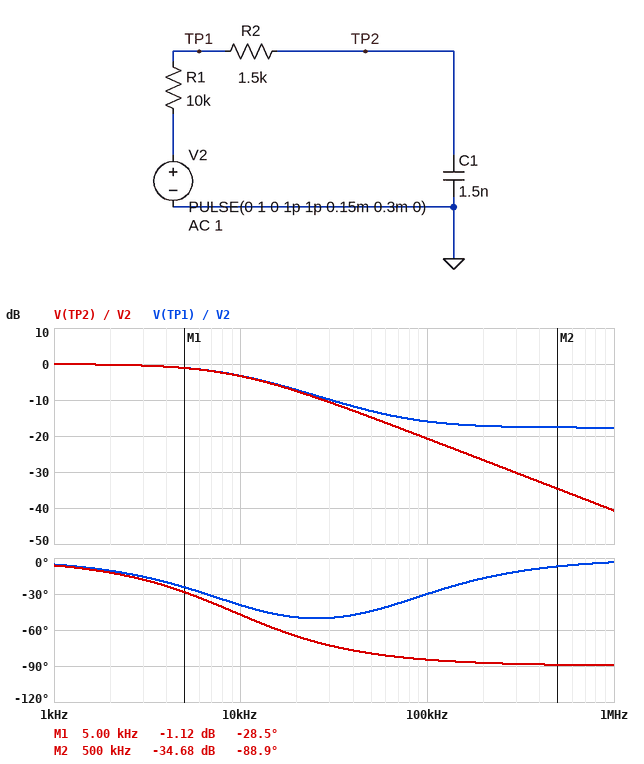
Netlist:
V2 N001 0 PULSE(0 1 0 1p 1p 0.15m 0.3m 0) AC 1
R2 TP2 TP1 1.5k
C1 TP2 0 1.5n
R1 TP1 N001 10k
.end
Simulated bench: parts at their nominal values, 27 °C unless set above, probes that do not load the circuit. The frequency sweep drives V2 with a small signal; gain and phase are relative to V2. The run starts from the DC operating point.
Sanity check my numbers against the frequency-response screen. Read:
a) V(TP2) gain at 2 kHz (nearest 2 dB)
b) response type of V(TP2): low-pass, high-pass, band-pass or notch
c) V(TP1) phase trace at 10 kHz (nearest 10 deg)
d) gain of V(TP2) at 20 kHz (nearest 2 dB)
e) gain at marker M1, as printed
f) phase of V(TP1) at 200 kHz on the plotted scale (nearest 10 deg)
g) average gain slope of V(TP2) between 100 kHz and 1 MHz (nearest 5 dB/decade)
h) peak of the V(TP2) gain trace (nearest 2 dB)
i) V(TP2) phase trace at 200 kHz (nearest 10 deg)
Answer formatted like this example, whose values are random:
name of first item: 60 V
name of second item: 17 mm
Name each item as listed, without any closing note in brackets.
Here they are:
V(TP2) gain at 2 kHz: 0 dB
response type of V(TP2): low-pass, high-pass, band-pass or notch: low-pass
V(TP1) phase trace at 10 kHz: -40 deg
gain of V(TP2) at 20 kHz: -8 dB
gain at marker M1, as printed: -1.12 dB
phase of V(TP1) at 200 kHz on the plotted scale: -20 deg
average gain slope of V(TP2) between 100 kHz and 1 MHz: -20 dB/decade
peak of the V(TP2) gain trace: 0 dB
V(TP2) phase trace at 200 kHz: -90 deg
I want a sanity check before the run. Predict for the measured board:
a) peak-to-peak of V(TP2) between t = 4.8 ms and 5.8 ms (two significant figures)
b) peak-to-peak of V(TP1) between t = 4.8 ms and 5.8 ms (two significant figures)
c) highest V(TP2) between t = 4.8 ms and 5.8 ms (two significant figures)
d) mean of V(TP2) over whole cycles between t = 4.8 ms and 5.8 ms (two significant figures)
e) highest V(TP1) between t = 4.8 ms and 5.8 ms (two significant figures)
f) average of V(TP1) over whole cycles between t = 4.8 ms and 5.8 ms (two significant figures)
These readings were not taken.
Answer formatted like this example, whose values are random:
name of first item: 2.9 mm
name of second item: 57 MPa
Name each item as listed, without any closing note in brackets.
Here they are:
peak-to-peak of V(TP2) between t = 4.8 ms and 5.8 ms: 1.0 V
peak-to-peak of V(TP1) between t = 4.8 ms and 5.8 ms: 1.0 V
highest V(TP2) between t = 4.8 ms and 5.8 ms: 1.0 V
mean of V(TP2) over whole cycles between t = 4.8 ms and 5.8 ms: 500 mV
highest V(TP1) between t = 4.8 ms and 5.8 ms: 1.0 V
average of V(TP1) over whole cycles between t = 4.8 ms and 5.8 ms: 500 mV
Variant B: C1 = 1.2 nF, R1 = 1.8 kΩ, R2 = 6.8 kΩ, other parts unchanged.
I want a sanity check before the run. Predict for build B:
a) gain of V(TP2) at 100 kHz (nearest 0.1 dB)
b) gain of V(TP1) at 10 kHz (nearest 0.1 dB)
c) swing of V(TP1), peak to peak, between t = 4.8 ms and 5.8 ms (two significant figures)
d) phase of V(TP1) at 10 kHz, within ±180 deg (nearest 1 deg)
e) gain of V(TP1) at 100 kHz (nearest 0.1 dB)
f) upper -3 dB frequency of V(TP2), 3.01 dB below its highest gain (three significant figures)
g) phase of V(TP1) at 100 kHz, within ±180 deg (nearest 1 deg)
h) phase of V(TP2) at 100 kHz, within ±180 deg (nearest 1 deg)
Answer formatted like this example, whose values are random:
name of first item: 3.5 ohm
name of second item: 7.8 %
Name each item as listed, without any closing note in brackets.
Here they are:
gain of V(TP2) at 100 kHz: -16.3 dB
gain of V(TP1) at 10 kHz: -0.5 dB
swing of V(TP1), peak to peak, between t = 4.8 ms and 5.8 ms: 1.0 V
phase of V(TP1) at 10 kHz, within ±180 deg: -6 deg
gain of V(TP1) at 100 kHz: -2.0 dB
upper -3 dB frequency of V(TP2), 3.01 dB below its highest gain: 15.4 kHz
phase of V(TP1) at 100 kHz, within ±180 deg: -2 deg
phase of V(TP2) at 100 kHz, within ±180 deg: -81 deg
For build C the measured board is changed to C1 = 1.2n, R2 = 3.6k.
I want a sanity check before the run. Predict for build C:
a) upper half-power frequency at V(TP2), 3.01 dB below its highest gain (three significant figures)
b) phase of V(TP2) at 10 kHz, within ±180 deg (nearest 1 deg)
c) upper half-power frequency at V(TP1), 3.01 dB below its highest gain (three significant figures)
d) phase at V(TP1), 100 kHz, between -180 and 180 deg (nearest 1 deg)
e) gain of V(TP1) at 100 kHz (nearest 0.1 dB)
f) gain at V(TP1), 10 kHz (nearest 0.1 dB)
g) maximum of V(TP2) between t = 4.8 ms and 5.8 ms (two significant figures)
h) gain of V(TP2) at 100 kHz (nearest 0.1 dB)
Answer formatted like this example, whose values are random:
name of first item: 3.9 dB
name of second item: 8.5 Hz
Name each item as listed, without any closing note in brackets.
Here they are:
upper half-power frequency at V(TP2), 3.01 dB below its highest gain: 9.75 kHz
phase of V(TP2) at 10 kHz, within ±180 deg: -46 deg
upper half-power frequency at V(TP1), 3.01 dB below its highest gain: 10.5 kHz
phase at V(TP1), 100 kHz, between -180 and 180 deg: -15 deg
gain of V(TP1) at 100 kHz: -11.0 dB
gain at V(TP1), 10 kHz: -2.8 dB
maximum of V(TP2) between t = 4.8 ms and 5.8 ms: 1.0 V
gain of V(TP2) at 100 kHz: -20.3 dB
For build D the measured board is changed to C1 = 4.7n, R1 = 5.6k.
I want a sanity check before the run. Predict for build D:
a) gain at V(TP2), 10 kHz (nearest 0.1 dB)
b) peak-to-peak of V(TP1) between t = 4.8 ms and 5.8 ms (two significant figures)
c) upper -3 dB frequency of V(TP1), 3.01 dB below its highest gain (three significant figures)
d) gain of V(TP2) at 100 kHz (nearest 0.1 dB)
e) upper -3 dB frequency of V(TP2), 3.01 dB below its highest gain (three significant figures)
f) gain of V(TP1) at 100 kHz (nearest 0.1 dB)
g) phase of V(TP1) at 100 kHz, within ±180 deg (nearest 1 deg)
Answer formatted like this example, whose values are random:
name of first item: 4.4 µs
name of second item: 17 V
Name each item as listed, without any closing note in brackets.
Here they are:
gain at V(TP2), 10 kHz: -7.3 dB
peak-to-peak of V(TP1) between t = 4.8 ms and 5.8 ms: 980 mV
upper -3 dB frequency of V(TP1), 3.01 dB below its highest gain: 5.00 kHz
gain of V(TP2) at 100 kHz: -26.4 dB
upper -3 dB frequency of V(TP2), 3.01 dB below its highest gain: 4.77 kHz
gain of V(TP1) at 100 kHz: -13.3 dB
phase of V(TP1) at 100 kHz, within ±180 deg: -10 deg
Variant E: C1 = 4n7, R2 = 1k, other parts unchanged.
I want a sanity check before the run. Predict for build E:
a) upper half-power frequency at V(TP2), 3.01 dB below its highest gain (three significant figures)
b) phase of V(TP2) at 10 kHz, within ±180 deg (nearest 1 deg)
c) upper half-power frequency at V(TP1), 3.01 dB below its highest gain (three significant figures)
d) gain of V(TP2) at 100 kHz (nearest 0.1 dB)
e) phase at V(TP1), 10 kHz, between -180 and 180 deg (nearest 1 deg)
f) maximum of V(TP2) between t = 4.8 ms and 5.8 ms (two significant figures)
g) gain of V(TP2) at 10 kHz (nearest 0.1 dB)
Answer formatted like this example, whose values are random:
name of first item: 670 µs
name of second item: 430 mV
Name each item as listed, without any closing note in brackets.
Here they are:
upper half-power frequency at V(TP2), 3.01 dB below its highest gain: 3.08 kHz
phase of V(TP2) at 10 kHz, within ±180 deg: -73 deg
upper half-power frequency at V(TP1), 3.01 dB below its highest gain: 3.10 kHz
gain of V(TP2) at 100 kHz: -30.2 dB
phase at V(TP1), 10 kHz, between -180 and 180 deg: -56 deg
maximum of V(TP2) between t = 4.8 ms and 5.8 ms: 950 mV
gain of V(TP2) at 10 kHz: -10.6 dB
